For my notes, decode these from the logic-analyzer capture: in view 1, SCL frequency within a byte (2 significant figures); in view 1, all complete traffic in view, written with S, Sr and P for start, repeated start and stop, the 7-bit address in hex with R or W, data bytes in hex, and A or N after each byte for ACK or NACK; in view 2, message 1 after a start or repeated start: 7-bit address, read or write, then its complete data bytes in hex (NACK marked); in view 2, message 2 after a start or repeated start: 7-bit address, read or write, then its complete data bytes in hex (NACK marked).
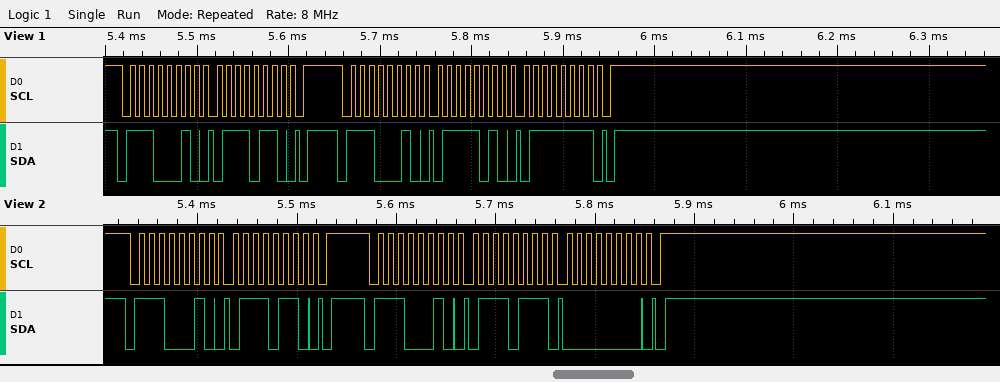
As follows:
100 kHz
S 71W A 76 A P S 71W A 7A A 7F A P
0x71 write: 76
0x71 write: 77 00
